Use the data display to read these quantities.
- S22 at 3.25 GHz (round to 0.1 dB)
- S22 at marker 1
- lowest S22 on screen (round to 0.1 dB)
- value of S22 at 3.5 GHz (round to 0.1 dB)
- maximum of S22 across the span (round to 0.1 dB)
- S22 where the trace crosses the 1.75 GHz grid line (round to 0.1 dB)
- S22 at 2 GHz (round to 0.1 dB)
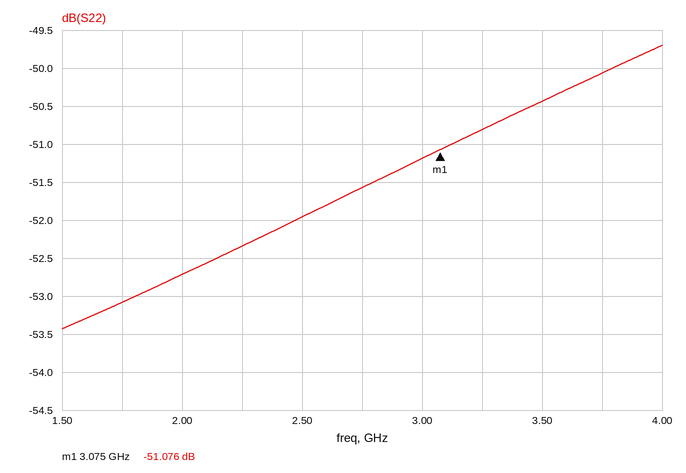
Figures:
-50.8 dB
-51.076 dB
-53.4 dB
-50.4 dB
-49.7 dB
-53.1 dB
-52.7 dB
